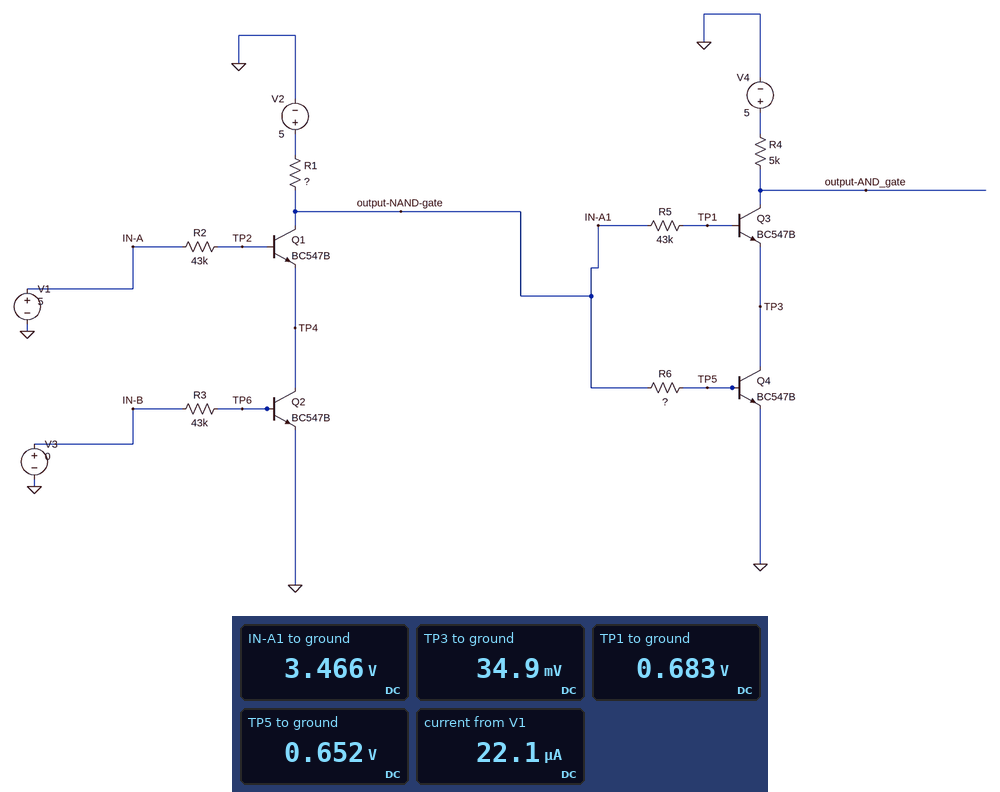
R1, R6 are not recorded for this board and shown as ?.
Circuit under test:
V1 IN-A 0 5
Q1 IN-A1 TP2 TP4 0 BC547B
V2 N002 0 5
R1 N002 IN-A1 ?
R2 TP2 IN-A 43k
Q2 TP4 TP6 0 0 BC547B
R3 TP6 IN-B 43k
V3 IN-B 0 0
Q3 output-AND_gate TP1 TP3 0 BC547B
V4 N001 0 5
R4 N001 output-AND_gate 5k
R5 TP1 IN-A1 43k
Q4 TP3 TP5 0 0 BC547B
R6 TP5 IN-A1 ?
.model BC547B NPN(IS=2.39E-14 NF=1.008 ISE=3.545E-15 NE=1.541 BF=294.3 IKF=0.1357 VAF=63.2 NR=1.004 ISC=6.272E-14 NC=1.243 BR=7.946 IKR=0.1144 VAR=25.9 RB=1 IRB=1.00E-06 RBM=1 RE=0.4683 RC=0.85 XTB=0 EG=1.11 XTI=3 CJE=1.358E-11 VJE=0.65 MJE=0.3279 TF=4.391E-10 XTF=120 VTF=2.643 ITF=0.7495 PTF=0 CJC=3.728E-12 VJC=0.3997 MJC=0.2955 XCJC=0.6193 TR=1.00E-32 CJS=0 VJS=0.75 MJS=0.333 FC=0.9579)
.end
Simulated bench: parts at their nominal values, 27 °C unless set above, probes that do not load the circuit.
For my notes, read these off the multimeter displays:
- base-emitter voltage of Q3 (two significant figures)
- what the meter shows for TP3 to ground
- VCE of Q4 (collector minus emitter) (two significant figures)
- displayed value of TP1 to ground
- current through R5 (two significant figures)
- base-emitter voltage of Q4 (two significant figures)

650 mV
34.9 mV
35 mV
0.683 V
65 µA
650 mV
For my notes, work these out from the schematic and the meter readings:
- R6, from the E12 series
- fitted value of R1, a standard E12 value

33 kΩ
12 kΩ
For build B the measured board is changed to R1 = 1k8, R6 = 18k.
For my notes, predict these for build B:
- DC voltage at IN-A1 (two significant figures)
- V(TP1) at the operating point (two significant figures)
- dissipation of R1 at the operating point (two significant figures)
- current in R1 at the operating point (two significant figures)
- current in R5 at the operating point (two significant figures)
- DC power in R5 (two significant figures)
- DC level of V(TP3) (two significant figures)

4.5 V
670 mV
160 µW
300 µA
88 µA
330 µW
22 mV
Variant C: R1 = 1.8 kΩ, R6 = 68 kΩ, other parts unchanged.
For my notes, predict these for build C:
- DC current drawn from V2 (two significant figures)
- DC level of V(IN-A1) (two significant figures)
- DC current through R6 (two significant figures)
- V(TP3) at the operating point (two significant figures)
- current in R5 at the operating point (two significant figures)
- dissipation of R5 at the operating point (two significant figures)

150 µA
4.7 V
60 µA
42 mV
94 µA
380 µW
